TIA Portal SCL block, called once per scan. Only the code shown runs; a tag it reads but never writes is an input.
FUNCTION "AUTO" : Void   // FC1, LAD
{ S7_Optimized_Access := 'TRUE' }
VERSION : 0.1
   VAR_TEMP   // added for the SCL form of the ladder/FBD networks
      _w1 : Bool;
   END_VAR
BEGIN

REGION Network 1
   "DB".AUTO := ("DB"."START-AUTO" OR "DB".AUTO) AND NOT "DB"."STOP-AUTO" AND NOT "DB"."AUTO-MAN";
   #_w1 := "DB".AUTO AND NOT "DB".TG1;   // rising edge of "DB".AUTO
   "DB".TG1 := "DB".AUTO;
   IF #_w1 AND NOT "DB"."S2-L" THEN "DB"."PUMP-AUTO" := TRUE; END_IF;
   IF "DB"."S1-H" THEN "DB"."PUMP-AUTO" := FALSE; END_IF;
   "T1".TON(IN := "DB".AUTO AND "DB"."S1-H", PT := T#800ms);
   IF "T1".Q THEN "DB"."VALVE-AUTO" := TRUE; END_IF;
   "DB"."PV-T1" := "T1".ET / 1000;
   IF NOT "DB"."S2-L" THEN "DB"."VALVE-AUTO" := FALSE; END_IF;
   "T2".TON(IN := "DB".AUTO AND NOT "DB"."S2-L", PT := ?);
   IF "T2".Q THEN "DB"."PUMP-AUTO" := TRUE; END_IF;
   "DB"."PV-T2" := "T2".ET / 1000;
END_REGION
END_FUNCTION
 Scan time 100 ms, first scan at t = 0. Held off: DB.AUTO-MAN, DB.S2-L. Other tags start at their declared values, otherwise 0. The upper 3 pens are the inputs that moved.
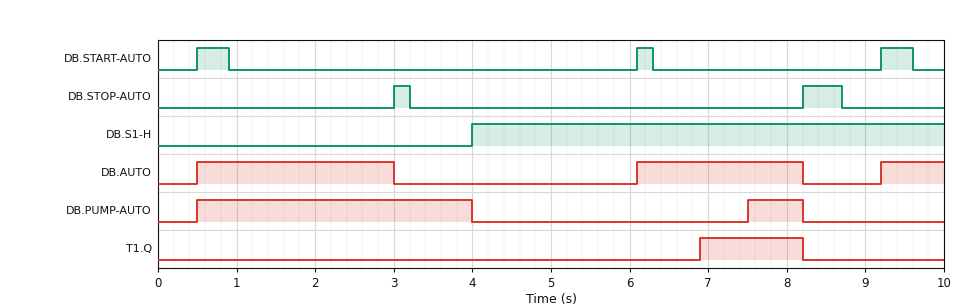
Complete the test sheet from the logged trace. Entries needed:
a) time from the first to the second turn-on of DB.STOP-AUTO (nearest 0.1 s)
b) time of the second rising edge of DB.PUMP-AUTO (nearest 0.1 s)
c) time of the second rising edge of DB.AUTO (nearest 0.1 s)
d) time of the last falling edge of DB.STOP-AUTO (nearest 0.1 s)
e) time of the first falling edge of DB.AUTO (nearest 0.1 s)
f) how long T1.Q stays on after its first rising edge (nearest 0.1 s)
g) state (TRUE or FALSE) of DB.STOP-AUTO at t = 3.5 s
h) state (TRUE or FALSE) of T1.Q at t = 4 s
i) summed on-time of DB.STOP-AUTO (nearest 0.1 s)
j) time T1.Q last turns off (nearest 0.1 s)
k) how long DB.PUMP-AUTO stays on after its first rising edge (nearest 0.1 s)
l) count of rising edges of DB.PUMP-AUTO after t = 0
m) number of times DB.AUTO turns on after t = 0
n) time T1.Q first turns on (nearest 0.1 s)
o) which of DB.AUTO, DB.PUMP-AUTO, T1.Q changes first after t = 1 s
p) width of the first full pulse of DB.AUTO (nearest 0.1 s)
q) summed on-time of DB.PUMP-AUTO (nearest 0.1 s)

5.2 s
7.5 s
6.1 s
8.7 s
3.0 s
1.3 s
FALSE
FALSE
0.7 s
8.2 s
3.5 s
2
3
6.9 s
DB.AUTO
2.5 s
4.2 s
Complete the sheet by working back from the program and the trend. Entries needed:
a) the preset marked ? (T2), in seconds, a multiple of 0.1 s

1.4 s
